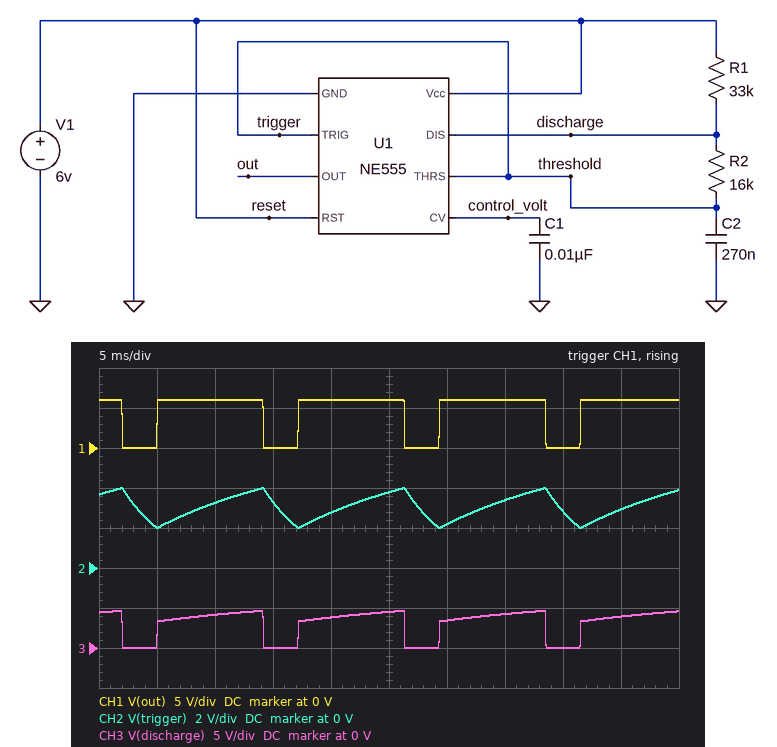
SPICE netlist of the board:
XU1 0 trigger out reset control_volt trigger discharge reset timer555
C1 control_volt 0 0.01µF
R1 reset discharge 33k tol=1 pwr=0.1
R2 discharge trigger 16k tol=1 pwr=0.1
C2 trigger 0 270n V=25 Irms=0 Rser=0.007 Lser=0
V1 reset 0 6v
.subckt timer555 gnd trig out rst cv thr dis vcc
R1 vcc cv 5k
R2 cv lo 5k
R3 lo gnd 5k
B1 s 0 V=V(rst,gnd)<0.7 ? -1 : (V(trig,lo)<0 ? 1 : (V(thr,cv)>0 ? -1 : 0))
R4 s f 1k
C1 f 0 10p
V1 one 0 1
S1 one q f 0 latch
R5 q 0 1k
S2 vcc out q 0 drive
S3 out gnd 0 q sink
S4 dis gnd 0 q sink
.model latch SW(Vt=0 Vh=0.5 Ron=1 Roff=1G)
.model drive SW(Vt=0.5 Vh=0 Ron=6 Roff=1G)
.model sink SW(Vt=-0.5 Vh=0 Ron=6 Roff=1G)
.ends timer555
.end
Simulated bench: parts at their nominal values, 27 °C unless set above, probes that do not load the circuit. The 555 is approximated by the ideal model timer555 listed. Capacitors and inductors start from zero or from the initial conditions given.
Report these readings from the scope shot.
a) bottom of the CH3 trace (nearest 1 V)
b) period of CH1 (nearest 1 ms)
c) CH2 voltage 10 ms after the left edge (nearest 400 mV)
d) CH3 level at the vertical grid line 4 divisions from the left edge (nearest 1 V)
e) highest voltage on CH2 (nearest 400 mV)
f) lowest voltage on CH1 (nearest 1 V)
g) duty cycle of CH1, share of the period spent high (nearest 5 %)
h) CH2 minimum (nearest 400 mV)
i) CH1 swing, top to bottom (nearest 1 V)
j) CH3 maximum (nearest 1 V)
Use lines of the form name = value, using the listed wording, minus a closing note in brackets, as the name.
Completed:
bottom of the CH3 trace = 0 V
period of CH1 = 12 ms
CH2 voltage 10 ms after the left edge = 3.2 V
CH3 level at the vertical grid line 4 divisions from the left edge = 4 V
highest voltage on CH2 = 4.0 V
lowest voltage on CH1 = 0 V
duty cycle of CH1, share of the period spent high = 75 %
CH2 minimum = 2.0 V
CH1 swing, top to bottom = 6 V
CH3 maximum = 5 V
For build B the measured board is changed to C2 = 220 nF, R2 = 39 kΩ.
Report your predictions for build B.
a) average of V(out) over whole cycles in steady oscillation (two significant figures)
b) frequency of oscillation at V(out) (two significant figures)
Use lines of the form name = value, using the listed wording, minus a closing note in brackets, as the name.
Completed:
average of V(out) over whole cycles in steady oscillation = 3.9 V
frequency of oscillation at V(out) = 59 Hz
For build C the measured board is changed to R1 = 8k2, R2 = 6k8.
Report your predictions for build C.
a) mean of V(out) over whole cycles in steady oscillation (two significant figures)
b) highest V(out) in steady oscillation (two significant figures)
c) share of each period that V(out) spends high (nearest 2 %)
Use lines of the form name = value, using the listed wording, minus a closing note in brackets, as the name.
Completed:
mean of V(out) over whole cycles in steady oscillation = 4.1 V
highest V(out) in steady oscillation = 6.0 V
share of each period that V(out) spends high = 68 %
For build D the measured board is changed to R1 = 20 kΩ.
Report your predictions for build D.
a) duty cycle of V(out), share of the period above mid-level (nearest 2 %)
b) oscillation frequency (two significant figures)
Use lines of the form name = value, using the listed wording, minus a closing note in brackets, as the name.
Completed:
duty cycle of V(out), share of the period above mid-level = 70 %
oscillation frequency = 100 Hz
